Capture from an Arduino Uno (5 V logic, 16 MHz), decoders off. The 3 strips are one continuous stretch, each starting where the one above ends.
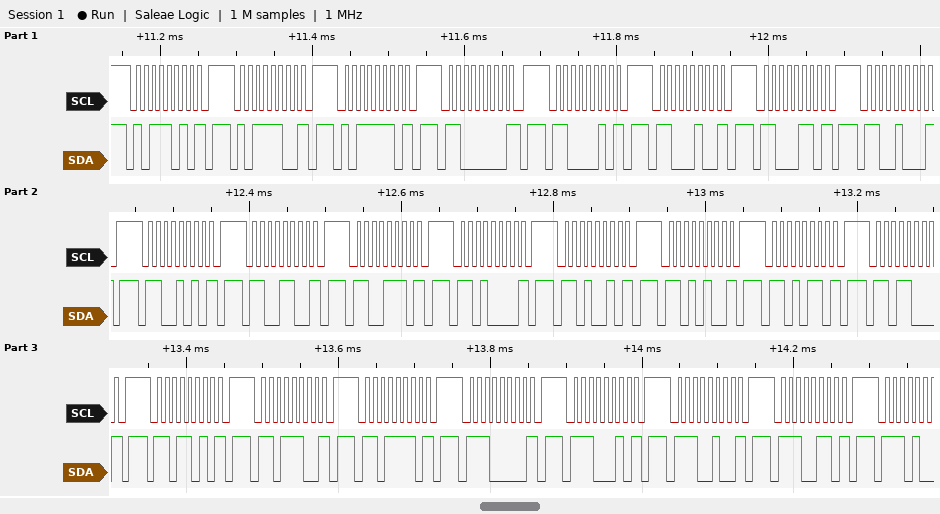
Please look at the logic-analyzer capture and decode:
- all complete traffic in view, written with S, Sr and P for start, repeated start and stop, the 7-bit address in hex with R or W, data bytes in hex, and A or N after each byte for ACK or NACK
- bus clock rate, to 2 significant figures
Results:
S 5DW N P S 5EW N P S 5FW N P S 60W N P S 61W N P S 62W N P S 63W N P S 64W N P S 65W N P S 66W N P S 67W N P S 68W N P S 69W N P S 6AW N P S 6BW N P S 6CW N P S 6DW N P S 6EW N P S 6FW N P S 70W N P S 71W N P S 72W N P S 73W N P
100 kHz
